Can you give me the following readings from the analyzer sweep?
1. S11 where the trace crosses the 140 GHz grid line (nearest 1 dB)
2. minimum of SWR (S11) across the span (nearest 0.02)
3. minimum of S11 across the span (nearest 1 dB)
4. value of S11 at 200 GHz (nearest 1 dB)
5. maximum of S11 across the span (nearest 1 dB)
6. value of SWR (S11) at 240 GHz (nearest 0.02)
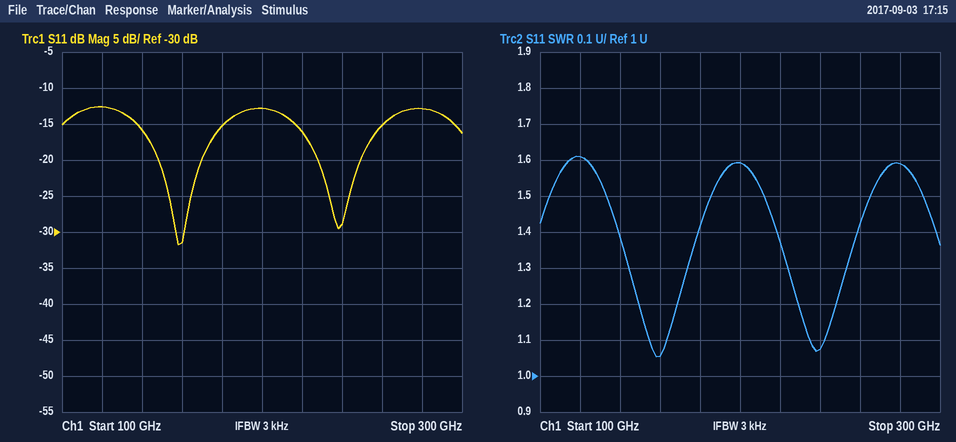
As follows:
-16 dB
1.06
-32 dB
-13 dB
-13 dB
1.08
